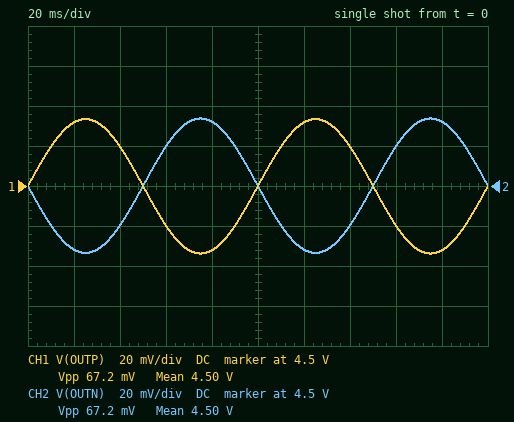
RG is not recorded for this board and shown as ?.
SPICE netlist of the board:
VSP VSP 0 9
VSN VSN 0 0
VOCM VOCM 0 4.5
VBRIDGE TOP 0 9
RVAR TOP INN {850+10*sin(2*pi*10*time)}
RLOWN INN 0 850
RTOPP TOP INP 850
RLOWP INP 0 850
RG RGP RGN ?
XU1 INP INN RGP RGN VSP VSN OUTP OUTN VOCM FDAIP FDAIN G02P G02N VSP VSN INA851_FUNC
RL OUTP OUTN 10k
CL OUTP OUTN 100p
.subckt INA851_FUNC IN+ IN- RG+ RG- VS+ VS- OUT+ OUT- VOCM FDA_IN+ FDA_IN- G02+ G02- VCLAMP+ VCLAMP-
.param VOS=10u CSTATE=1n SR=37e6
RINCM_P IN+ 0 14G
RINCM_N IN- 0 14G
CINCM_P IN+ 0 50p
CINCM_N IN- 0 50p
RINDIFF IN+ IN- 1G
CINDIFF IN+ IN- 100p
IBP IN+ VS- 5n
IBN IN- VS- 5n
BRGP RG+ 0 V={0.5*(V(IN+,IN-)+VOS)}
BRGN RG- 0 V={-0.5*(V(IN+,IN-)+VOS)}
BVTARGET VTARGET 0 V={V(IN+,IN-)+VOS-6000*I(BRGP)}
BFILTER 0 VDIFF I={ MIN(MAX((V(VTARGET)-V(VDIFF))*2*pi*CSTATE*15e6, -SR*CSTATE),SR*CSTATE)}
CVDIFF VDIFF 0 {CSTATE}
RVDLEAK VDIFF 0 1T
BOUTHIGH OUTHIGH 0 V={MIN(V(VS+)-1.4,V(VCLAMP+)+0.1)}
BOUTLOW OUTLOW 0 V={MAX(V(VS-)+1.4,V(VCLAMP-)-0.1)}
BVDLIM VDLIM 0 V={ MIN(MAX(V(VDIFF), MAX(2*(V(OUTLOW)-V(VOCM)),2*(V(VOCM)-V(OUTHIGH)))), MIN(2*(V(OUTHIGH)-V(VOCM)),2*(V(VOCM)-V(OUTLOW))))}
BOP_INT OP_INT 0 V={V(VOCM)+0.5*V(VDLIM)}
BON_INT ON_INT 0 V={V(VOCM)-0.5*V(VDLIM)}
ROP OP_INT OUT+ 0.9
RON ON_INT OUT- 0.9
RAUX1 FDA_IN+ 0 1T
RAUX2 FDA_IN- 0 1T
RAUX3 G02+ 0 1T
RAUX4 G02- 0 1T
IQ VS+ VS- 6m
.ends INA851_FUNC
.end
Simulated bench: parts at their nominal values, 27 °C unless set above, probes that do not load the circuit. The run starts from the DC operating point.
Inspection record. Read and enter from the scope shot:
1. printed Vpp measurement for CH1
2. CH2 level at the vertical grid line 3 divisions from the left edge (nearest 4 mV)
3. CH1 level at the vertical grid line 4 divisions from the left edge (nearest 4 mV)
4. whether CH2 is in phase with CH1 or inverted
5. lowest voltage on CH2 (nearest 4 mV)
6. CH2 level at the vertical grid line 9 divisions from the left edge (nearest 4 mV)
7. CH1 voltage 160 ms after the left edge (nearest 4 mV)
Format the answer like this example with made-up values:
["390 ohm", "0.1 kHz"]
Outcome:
["67.2 mV", "4.520 V", "4.468 V", "inverted", "4.468 V", "4.532 V", "4.480 V"]
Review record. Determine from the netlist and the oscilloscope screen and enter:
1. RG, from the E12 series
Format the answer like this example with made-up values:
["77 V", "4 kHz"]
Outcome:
["3.9 kΩ"]
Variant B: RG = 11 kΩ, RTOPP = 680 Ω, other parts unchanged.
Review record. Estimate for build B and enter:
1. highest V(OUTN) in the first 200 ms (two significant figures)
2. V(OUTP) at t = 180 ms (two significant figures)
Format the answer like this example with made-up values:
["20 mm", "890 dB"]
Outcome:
["4.1 V", "4.9 V"]
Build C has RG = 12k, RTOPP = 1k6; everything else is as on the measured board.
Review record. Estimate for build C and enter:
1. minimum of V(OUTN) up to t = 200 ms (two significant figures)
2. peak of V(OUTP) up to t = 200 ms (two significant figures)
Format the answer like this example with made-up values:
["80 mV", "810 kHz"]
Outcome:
["5.5 V", "3.5 V"]
